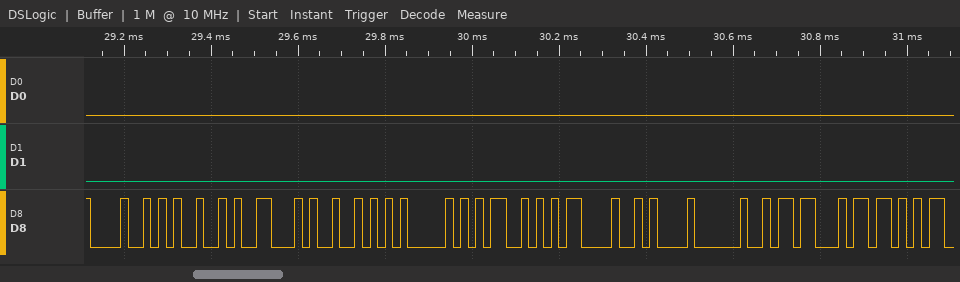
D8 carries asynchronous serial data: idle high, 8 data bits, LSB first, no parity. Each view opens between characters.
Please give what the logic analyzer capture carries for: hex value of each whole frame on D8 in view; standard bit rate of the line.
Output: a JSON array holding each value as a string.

["48, 49, 46, 52, 41, 4D, 0D, 0A, 20, 1B, 5B", "57600 baud"]
